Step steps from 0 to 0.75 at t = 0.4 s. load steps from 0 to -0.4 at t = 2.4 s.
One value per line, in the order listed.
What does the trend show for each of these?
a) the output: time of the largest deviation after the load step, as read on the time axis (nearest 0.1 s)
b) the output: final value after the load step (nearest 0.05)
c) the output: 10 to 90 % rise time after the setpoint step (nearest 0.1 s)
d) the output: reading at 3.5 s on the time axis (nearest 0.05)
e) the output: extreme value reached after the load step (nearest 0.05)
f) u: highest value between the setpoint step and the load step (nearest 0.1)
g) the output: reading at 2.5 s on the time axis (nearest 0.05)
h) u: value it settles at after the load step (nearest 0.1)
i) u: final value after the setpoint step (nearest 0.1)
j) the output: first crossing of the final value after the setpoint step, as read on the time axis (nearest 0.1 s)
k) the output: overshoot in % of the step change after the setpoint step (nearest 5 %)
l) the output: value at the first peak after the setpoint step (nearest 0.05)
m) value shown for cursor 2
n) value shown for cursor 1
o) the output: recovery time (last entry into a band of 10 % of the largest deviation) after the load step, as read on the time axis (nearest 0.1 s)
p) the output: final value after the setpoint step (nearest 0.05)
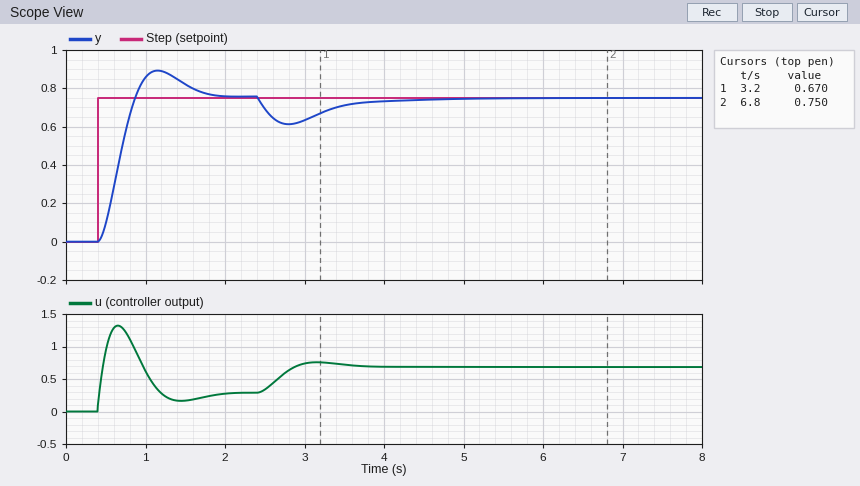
2.8 s
0.75
0.3 s
0.70
0.60
1.3
0.70
0.7
0.3
0.9 s
20 %
0.90
0.750
0.670
4.2 s
0.75
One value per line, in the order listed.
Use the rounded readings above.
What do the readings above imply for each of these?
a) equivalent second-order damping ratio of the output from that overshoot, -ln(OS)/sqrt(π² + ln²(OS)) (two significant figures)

0.46
